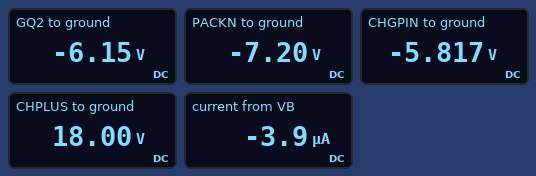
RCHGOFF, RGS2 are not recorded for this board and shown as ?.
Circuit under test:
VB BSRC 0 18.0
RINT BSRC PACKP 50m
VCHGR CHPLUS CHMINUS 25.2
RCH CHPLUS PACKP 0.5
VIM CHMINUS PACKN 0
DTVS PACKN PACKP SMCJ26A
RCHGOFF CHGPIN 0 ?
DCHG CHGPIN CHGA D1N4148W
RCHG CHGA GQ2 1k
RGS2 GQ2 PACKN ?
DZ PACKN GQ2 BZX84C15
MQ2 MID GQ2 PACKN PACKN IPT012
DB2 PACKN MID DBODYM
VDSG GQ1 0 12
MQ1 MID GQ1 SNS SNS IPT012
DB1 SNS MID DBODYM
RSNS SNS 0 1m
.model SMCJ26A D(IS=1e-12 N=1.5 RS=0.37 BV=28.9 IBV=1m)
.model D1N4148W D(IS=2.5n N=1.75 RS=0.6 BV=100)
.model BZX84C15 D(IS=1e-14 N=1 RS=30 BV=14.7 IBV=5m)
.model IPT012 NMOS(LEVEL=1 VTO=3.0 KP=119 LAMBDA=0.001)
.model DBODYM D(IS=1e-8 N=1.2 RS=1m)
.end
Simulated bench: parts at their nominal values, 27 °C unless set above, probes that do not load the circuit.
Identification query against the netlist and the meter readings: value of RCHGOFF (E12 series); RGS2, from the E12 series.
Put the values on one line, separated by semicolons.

1.5 MΩ; 270 kΩ
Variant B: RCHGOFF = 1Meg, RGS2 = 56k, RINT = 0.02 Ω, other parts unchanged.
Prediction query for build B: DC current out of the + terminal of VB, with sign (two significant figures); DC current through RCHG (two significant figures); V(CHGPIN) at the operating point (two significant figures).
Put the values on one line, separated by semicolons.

-6.5 µA; 6.5 µA; -6.5 V
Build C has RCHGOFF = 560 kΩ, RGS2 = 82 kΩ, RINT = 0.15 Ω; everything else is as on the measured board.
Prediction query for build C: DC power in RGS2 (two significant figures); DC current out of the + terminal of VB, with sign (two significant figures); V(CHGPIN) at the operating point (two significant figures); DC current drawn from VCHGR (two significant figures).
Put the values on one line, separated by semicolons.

9.2 µW; -11 µA; -5.9 V; 11 µA
